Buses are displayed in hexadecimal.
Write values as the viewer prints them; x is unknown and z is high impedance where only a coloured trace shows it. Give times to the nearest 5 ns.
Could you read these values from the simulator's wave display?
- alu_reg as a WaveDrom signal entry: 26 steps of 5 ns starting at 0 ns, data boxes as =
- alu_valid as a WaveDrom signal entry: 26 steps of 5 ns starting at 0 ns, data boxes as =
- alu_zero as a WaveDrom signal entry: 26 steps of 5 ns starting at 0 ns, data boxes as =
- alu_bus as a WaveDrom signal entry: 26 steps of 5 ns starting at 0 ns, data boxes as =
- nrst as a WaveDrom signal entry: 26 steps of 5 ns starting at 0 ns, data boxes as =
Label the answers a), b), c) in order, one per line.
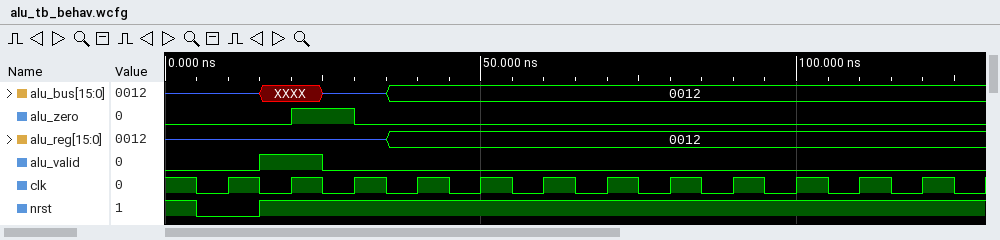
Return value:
a) {name: 'alu_reg', wave: 'z......=..................', data: '0012'}
b) {name: 'alu_valid', wave: '0..1.0....................'}
c) {name: 'alu_zero', wave: '0...1.0...................'}
d) {name: 'alu_bus', wave: 'z..x.z.=..................', data: '0012'}
e) {name: 'nrst', wave: '10.1......................'}
